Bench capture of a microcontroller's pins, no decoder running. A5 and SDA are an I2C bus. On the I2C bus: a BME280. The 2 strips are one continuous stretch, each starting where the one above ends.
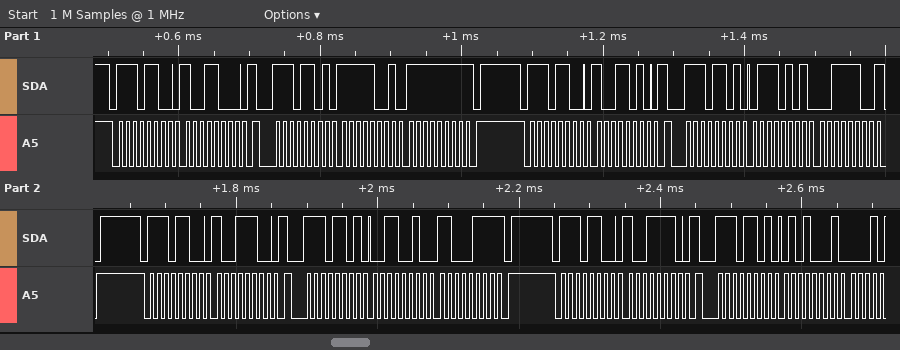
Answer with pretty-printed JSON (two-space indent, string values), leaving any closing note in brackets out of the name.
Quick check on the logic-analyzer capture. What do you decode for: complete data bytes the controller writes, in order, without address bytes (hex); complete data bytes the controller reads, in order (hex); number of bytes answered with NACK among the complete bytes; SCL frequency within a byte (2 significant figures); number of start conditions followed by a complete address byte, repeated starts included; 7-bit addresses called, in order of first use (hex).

{
  "complete data bytes the controller writes, in order, without address bytes": "98 9A 9C 9E",
  "complete data bytes the controller reads, in order": "F9 FF 75 3C 32 C7 51",
  "number of bytes answered with NACK among the complete bytes": "3",
  "SCL frequency within a byte": "100 kHz",
  "number of start conditions followed by a complete address byte, repeated starts included": "8",
  "7-bit addresses called, in order of first use": "0x76"
}
